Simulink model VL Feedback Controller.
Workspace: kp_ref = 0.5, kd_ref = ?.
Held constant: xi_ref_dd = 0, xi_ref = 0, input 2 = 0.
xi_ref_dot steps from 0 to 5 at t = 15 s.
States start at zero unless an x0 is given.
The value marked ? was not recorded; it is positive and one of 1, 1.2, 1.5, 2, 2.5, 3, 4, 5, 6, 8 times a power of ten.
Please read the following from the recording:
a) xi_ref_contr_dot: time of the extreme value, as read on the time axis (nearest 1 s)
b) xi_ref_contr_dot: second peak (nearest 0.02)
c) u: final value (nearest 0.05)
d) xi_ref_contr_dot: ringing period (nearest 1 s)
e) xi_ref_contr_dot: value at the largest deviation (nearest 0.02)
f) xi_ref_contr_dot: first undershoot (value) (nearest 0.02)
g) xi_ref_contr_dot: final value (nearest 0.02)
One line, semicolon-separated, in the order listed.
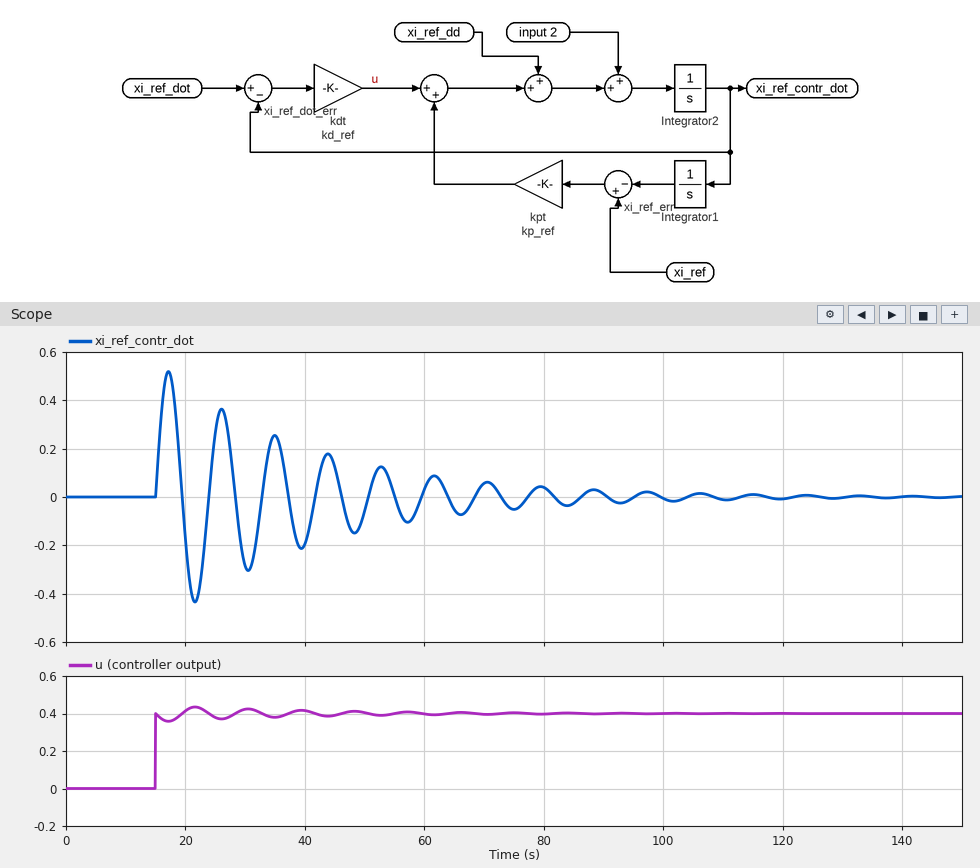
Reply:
17 s; 0.36; 0.40; 9 s; 0.52; -0.44; 0.00
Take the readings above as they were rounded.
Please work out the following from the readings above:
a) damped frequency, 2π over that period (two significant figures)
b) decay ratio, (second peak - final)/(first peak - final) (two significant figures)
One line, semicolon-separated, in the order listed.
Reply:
0.70 rad/s; 0.69
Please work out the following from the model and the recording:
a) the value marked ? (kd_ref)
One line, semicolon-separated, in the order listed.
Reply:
0.08
